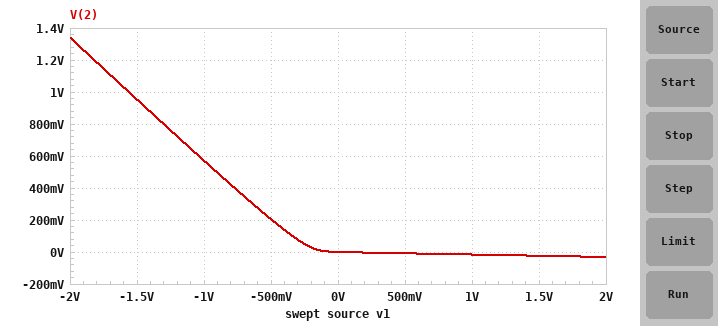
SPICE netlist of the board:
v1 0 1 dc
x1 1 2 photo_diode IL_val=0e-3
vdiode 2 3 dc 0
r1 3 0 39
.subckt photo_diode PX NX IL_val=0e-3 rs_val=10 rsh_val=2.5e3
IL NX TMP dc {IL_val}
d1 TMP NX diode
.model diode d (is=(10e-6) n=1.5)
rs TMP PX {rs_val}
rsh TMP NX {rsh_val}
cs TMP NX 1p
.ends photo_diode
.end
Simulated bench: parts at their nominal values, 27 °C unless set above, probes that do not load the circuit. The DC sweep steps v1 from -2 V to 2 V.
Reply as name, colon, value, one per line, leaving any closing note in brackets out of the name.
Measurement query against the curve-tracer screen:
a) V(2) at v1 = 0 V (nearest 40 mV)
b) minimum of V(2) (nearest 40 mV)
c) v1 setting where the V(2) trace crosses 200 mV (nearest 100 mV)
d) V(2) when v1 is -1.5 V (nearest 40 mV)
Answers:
V(2) at v1 = 0 V: 0 V
minimum of V(2): -40 mV
v1 setting where the V(2) trace crosses 200 mV: -500 mV
V(2) when v1 is -1.5 V: 960 mV
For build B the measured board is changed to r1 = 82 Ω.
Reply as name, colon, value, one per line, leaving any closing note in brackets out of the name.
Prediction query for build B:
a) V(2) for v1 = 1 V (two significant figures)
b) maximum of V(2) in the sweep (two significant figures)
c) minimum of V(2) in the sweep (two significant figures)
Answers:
V(2) for v1 = 1 V: -32 mV
maximum of V(2) in the sweep: 1.5 V
minimum of V(2) in the sweep: -64 mV
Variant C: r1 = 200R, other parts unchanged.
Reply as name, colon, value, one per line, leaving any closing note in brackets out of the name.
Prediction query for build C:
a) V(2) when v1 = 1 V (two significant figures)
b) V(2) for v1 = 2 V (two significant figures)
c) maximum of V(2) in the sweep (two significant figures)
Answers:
V(2) when v1 = 1 V: -76 mV
V(2) for v1 = 2 V: -150 mV
maximum of V(2) in the sweep: 1.7 V
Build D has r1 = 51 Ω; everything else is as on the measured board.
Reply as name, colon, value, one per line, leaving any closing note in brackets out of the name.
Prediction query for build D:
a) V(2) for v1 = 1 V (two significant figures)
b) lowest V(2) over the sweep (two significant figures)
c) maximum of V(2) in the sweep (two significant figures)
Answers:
V(2) for v1 = 1 V: -20 mV
lowest V(2) over the sweep: -40 mV
maximum of V(2) in the sweep: 1.4 V
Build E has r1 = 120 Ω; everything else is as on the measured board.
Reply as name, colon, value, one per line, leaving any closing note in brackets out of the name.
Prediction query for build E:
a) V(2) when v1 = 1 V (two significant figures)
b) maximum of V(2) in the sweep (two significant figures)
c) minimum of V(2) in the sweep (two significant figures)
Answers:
V(2) when v1 = 1 V: -47 mV
maximum of V(2) in the sweep: 1.6 V
minimum of V(2) in the sweep: -92 mV
